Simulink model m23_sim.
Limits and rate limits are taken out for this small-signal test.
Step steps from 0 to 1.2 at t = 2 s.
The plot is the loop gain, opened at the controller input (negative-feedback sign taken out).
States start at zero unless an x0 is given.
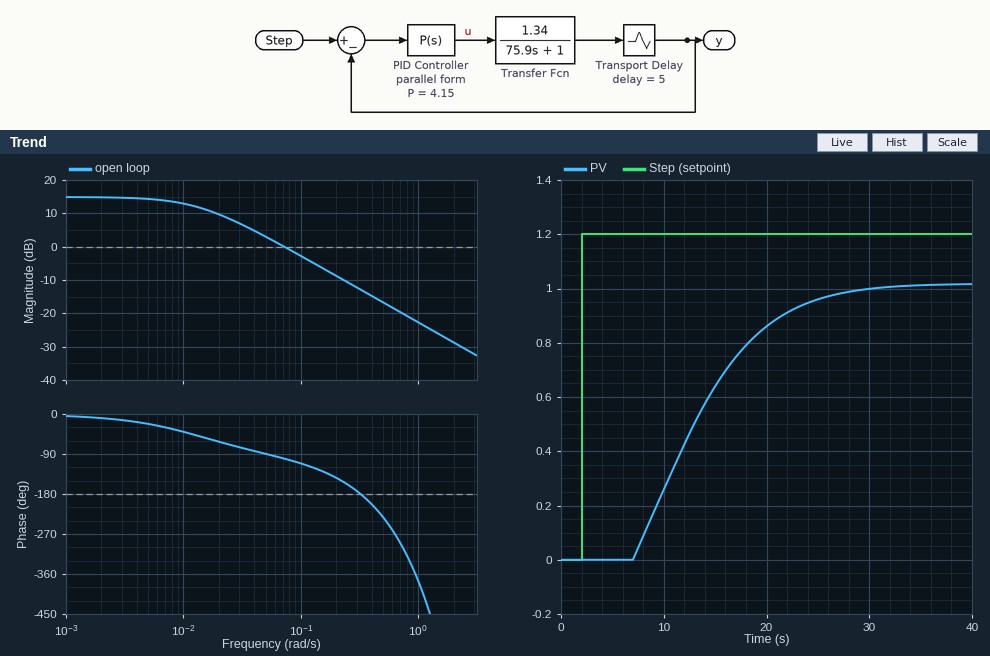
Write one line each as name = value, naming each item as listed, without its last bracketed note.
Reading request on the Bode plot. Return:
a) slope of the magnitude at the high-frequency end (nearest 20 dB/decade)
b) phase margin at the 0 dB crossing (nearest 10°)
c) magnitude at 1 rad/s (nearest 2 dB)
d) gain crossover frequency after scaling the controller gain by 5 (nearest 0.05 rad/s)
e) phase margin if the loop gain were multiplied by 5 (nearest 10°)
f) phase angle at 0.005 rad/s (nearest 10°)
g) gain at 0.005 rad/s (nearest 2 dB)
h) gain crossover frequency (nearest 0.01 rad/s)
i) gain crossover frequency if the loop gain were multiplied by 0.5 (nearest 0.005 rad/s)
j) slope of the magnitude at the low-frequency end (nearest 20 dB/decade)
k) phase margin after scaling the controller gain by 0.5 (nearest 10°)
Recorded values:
slope of the magnitude at the high-frequency end = -20 dB/decade
phase margin at the 0 dB crossing = 80°
magnitude at 1 rad/s = -22 dB
gain crossover frequency after scaling the controller gain by 5 = 0.35 rad/s
phase margin if the loop gain were multiplied by 5 = -10°
phase angle at 0.005 rad/s = -20°
gain at 0.005 rad/s = 14 dB
gain crossover frequency = 0.07 rad/s
gain crossover frequency if the loop gain were multiplied by 0.5 = 0.035 rad/s
slope of the magnitude at the low-frequency end = 0 dB/decade
phase margin after scaling the controller gain by 0.5 = 100°
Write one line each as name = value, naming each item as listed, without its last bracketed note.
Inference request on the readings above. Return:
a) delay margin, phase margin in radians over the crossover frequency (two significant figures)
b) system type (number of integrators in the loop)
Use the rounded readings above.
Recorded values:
delay margin, phase margin in radians over the crossover frequency = 20 s
system type = 0
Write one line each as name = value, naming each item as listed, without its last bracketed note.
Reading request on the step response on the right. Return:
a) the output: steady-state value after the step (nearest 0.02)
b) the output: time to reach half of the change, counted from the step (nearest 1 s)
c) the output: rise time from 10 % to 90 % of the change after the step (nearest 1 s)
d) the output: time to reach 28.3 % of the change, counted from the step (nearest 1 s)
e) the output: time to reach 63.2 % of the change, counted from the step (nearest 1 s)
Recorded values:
the output: steady-state value after the step = 1.02
the output: time to reach half of the change, counted from the step = 11 s
the output: rise time from 10 % to 90 % of the change after the step = 14 s
the output: time to reach 28.3 % of the change, counted from the step = 8 s
the output: time to reach 63.2 % of the change, counted from the step = 13 s
